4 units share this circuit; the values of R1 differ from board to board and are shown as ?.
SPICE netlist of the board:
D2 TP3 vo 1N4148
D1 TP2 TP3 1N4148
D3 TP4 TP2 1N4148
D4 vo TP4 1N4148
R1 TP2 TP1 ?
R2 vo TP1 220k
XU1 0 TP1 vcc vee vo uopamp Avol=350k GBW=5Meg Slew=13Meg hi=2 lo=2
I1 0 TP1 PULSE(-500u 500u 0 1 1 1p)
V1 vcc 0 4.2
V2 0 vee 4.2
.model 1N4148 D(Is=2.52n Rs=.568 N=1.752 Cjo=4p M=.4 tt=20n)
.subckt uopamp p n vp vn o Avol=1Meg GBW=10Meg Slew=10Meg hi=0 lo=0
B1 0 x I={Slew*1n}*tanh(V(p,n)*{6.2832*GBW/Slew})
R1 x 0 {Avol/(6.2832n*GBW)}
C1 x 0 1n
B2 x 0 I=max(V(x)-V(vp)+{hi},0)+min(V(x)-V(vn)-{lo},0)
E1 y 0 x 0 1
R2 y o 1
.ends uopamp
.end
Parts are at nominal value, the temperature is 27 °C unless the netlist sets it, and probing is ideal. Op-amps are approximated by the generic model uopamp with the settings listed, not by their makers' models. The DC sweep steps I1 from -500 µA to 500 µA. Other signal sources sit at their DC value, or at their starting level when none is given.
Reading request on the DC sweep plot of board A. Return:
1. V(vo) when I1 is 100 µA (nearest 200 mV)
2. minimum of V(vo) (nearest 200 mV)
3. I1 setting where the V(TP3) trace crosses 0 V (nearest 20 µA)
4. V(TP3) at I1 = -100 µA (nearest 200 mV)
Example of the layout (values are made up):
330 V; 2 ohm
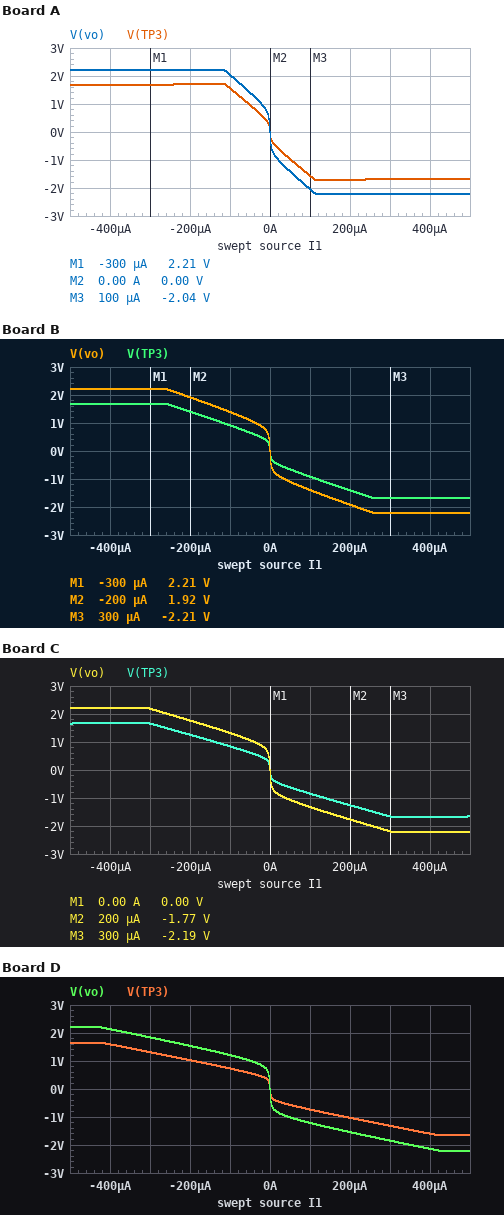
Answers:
-2.0 V; -2.2 V; 0 A; 1.6 V
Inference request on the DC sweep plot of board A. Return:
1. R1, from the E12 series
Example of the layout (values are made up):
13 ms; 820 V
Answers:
12 kΩ
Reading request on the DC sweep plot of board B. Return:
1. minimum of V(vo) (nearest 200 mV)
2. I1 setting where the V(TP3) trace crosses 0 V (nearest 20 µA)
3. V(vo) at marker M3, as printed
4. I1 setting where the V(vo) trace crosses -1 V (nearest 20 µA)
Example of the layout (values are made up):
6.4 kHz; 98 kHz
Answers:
-2.2 V; 0 A; -2.21 V; 40 µA
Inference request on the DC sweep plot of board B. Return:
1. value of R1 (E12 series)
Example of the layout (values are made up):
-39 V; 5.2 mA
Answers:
4.7 kΩ
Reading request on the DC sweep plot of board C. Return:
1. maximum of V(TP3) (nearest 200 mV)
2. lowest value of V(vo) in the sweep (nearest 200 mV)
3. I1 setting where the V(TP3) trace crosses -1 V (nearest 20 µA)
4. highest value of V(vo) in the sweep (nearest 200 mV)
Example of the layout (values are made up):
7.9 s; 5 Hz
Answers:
1.6 V; -2.2 V; 140 µA; 2.2 V
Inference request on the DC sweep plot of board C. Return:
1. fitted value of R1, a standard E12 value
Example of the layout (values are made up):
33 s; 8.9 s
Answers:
3.9 kΩ
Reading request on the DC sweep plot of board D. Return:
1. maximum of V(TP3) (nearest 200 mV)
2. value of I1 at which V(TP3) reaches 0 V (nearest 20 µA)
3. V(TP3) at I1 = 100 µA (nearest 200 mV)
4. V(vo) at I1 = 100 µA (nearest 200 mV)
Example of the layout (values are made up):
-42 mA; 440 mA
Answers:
1.6 V; 0 A; -800 mV; -1.2 V
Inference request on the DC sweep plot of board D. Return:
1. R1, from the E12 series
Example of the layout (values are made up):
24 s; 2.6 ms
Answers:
2.7 kΩ
